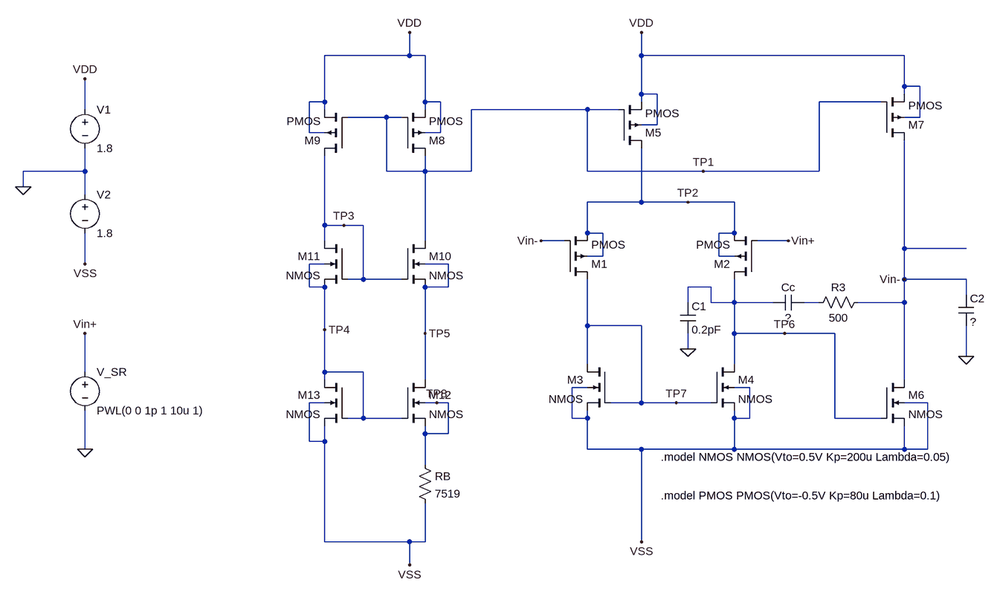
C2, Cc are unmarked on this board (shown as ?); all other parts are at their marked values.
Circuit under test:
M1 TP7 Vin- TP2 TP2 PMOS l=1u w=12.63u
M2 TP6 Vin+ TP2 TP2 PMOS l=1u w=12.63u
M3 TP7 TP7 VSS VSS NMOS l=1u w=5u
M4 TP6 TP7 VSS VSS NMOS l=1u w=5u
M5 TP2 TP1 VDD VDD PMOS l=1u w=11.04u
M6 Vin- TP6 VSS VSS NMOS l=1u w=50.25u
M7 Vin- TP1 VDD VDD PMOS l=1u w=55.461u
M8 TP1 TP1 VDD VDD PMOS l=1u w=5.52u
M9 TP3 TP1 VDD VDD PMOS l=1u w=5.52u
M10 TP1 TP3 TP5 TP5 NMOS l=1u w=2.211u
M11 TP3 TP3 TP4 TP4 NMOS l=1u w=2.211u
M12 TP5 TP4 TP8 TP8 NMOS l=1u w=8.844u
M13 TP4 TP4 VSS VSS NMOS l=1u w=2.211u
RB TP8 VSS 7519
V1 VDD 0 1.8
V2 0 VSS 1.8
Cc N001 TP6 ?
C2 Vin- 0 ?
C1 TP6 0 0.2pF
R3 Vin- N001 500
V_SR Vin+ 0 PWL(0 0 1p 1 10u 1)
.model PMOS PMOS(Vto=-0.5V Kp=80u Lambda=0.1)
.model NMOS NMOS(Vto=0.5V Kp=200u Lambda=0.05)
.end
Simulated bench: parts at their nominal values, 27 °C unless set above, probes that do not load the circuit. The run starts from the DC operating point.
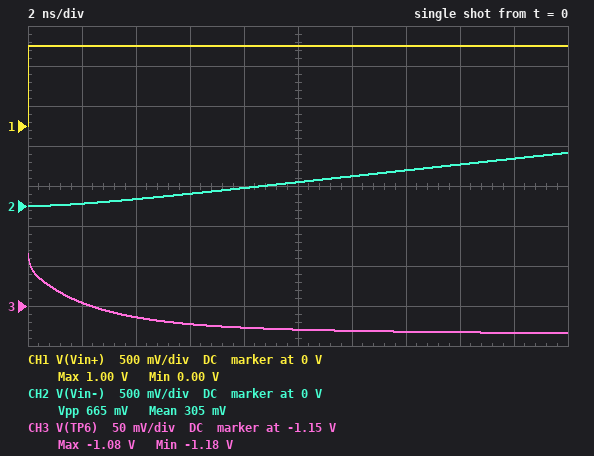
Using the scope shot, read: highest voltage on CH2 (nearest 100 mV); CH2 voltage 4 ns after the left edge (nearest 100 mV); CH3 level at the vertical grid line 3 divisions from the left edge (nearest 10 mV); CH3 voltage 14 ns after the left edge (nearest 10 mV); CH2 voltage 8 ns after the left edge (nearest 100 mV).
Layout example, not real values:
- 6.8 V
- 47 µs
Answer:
- 700 mV
- 100 mV
- -1.17 V
- -1.18 V
- 200 mV
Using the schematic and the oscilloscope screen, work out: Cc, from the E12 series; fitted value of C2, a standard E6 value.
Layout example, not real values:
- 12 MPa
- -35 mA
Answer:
- 1.2 pF
- 3.3 pF
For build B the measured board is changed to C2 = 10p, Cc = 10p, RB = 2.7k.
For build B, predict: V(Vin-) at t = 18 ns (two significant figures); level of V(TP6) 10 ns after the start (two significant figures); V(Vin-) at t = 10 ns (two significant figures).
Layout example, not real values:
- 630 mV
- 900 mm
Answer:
- 400 mV
- -870 mV
- 250 mV
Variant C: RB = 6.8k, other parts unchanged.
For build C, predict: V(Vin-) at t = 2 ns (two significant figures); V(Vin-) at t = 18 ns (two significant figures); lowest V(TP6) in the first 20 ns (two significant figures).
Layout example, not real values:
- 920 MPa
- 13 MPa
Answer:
- 38 mV
- 710 mV
- -1.2 V
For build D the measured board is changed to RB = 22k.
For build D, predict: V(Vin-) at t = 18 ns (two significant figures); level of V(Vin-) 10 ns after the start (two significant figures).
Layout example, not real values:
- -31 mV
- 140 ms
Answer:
- 60 mV
- 24 mV
